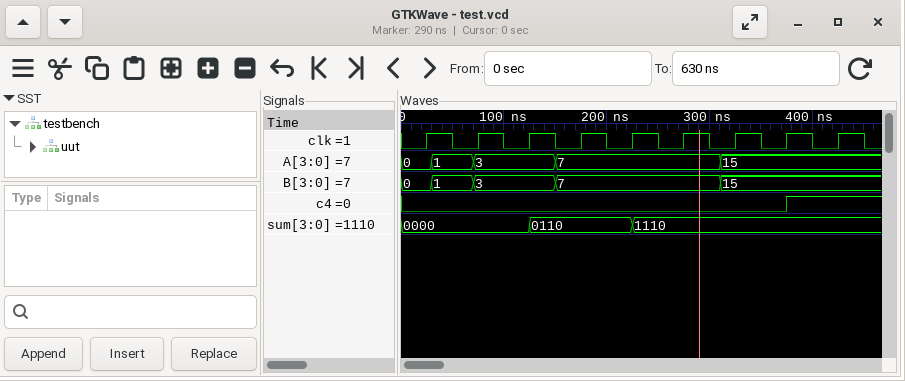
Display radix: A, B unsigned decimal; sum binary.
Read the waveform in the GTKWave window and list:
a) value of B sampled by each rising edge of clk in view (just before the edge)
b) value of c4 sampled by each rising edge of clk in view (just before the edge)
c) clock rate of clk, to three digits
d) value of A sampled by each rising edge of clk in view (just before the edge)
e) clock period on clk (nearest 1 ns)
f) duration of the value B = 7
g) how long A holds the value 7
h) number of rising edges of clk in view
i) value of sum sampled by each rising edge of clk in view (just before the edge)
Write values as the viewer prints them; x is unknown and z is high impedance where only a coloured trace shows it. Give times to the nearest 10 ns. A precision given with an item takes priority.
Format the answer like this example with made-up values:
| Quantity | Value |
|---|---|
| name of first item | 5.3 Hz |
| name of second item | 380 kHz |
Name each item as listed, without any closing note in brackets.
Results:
| Quantity | Value |
|---|---|
| value of B sampled by each rising edge of clk in view | 0, 3, 3, 7, 7, 7, 15, 15, 15 |
| value of c4 sampled by each rising edge of clk in view | 0 0 0 0 0 0 0 0 1 |
| clock rate of clk, to three digits | 20.0 MHz |
| value of A sampled by each rising edge of clk in view | 0, 3, 3, 7, 7, 7, 15, 15, 15 |
| clock period on clk | 50 ns |
| duration of the value B = 7 | 160 ns |
| how long A holds the value 7 | 160 ns |
| number of rising edges of clk in view | 9 |
| value of sum sampled by each rising edge of clk in view | 0000, 0000, 0000, 0110, 0110, 1110, 1110, 1110, 1110 |
